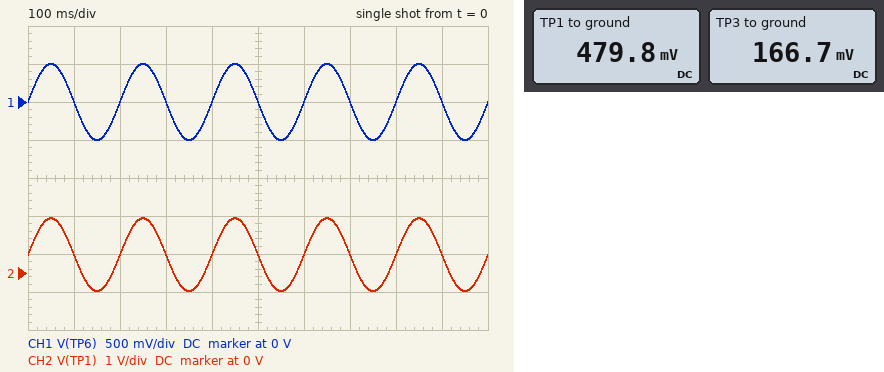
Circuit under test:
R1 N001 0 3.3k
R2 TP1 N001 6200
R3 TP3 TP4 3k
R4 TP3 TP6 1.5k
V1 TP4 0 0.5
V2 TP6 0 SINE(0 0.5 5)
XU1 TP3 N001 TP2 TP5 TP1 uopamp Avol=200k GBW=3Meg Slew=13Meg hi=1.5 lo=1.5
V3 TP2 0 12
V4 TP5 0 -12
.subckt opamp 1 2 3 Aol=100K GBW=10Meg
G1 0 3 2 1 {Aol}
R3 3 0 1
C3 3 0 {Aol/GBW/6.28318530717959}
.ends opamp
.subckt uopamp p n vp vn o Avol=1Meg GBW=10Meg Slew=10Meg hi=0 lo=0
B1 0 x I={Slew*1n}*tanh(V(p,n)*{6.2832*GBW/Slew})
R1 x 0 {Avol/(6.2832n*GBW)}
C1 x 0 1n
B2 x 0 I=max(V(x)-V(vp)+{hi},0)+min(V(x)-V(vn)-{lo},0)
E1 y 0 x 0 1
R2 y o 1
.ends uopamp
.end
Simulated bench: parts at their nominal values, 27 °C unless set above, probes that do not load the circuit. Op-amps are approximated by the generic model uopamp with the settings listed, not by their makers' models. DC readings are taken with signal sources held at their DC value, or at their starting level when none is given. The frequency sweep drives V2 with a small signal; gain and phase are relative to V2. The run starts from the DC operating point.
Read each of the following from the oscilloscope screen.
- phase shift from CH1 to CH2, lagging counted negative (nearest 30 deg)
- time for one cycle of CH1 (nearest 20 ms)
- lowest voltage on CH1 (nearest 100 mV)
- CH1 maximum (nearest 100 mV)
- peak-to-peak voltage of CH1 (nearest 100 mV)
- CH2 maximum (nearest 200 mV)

0 deg
200 ms
-500 mV
500 mV
1.0 V
1.4 V
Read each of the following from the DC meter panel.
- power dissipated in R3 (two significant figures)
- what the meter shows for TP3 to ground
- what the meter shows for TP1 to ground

37 µW
166.7 mV
479.8 mV
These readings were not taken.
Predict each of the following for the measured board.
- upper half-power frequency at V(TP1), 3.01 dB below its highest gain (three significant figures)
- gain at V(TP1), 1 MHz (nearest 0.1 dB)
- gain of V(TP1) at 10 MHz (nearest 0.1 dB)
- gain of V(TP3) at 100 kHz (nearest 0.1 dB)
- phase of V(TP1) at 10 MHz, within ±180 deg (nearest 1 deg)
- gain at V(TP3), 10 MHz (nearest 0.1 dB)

1.04 MHz
2.8 dB
-14.0 dB
-3.5 dB
-84 deg
-3.5 dB
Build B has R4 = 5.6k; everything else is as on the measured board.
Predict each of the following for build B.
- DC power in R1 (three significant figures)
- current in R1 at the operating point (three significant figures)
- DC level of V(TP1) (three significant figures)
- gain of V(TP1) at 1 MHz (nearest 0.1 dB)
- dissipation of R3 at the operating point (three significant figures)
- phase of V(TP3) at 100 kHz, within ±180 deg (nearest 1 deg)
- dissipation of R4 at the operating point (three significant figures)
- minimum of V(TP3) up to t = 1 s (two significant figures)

32.1 µW
98.7 µA
937 mV
-2.8 dB
10.1 µW
0 deg
18.9 µW
150 mV
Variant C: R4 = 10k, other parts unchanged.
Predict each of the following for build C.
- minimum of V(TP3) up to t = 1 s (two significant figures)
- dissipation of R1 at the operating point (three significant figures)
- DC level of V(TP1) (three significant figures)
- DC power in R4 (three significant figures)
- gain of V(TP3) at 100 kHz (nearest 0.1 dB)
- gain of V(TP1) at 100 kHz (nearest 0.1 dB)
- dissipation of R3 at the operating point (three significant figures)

270 mV
44.8 µW
1.11 V
14.8 µW
-12.7 dB
-3.6 dB
4.44 µW
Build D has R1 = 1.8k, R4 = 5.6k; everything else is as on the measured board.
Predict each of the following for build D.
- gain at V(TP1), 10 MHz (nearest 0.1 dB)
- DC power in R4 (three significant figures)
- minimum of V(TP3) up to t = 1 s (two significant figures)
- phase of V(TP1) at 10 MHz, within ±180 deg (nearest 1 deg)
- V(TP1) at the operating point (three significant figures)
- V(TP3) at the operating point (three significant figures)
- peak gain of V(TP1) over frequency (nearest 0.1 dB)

-19.6 dB
18.9 µW
150 mV
-86 deg
1.45 V
326 mV
3.8 dB
